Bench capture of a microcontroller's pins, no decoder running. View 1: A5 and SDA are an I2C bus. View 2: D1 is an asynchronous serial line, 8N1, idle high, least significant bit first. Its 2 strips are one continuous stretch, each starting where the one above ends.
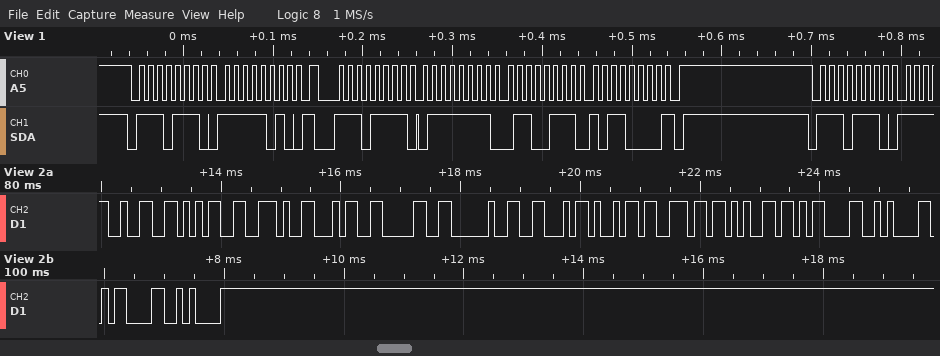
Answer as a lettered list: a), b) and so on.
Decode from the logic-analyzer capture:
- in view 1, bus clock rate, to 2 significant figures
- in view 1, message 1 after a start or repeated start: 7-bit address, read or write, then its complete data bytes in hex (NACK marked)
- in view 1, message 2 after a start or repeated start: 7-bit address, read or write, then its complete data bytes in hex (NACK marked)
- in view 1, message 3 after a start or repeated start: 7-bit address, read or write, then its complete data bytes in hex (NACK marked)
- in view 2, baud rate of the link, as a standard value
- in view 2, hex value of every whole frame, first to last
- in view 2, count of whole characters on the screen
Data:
a) 100 kHz
b) 0x77 write: FA
c) 0x77 read: 7F 67 B0 NACK
d) 0x77 write
e) 9600 baud
f) 0x32 0x35 0x2E 0x34 0x30 0x20 0x46 0x69 0x6E 0x65 0x0D 0x0A 0x0D 0x0A
g) 14
